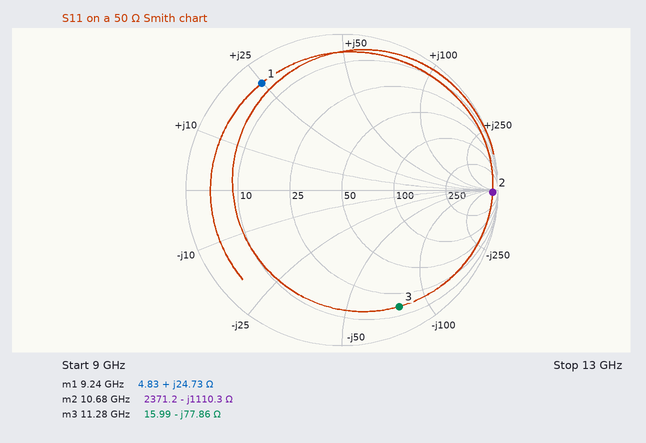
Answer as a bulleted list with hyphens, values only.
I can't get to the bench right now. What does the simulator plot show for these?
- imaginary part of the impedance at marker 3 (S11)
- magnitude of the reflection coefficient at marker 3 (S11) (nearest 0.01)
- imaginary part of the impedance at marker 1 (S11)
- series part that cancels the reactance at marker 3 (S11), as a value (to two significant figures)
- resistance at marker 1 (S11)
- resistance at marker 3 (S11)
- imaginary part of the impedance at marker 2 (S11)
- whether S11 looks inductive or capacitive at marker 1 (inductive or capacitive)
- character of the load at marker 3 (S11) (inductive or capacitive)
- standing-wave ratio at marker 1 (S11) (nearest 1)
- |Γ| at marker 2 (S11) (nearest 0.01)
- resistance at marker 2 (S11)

- -77.86 Ω
- 0.83
- +24.73 Ω
- 1.1 nH
- 4.83 Ω
- 15.99 Ω
- -1110.3 Ω
- inductive
- capacitive
- 13
- 0.97
- 2371.2 Ω
